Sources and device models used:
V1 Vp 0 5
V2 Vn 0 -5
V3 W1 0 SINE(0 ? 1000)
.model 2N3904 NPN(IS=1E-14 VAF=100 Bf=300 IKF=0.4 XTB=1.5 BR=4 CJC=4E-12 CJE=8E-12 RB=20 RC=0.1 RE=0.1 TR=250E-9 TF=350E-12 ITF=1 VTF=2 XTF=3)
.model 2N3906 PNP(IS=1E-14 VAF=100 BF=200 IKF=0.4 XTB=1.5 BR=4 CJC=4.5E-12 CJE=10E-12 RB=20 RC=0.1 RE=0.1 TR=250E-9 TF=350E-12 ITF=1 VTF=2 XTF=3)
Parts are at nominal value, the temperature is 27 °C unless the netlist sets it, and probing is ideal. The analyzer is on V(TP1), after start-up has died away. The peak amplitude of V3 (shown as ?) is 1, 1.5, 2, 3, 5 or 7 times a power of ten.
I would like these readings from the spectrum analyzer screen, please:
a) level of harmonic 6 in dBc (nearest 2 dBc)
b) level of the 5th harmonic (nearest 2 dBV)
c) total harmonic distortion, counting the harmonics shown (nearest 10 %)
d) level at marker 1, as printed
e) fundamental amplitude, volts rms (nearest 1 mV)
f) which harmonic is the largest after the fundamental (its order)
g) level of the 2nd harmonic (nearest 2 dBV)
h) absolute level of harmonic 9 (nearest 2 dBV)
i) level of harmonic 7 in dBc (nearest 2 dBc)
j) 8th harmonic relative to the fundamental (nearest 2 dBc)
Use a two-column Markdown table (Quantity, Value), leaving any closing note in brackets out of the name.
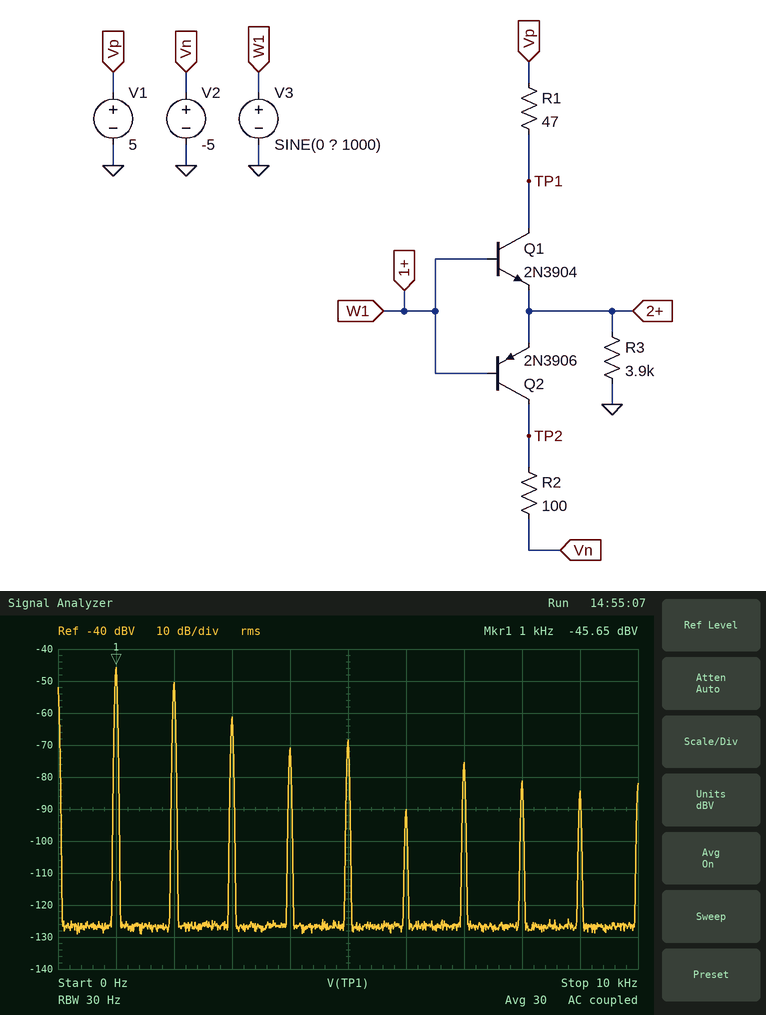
| Quantity | Value |
|---|---|
| level of harmonic 6 in dBc | -44 dBc |
| level of the 5th harmonic | -68 dBV |
| total harmonic distortion, counting the harmonics shown | 60 % |
| level at marker 1, as printed | -45.65 dBV |
| fundamental amplitude, volts rms | 5 mV |
| which harmonic is the largest after the fundamental | 2 |
| level of the 2nd harmonic | -50 dBV |
| absolute level of harmonic 9 | -84 dBV |
| level of harmonic 7 in dBc | -30 dBc |
| 8th harmonic relative to the fundamental | -36 dBc |
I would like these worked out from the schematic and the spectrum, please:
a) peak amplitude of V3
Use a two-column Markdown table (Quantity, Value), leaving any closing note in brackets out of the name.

| Quantity | Value |
|---|---|
| peak amplitude of V3 | 2 V |
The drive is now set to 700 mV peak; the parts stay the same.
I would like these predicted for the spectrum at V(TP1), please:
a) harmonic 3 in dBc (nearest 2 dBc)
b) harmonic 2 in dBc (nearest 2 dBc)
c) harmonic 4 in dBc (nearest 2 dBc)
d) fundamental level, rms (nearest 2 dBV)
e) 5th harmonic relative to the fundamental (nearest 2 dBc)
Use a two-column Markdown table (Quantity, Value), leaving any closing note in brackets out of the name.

| Quantity | Value |
|---|---|
| harmonic 3 in dBc | -4 dBc |
| harmonic 2 in dBc | -2 dBc |
| harmonic 4 in dBc | -8 dBc |
| fundamental level, rms | -70 dBV |
| 5th harmonic relative to the fundamental | -16 dBc |
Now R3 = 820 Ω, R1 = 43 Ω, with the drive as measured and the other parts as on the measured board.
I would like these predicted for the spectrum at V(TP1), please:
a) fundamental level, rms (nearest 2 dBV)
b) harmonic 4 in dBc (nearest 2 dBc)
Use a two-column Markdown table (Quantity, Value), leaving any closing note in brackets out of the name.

| Quantity | Value |
|---|---|
| fundamental level, rms | -34 dBV |
| harmonic 4 in dBc | -26 dBc |
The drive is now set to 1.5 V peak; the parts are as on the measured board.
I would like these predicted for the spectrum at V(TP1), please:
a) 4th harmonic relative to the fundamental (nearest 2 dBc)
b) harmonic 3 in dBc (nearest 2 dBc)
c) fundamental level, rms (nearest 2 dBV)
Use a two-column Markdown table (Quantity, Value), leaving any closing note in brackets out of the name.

| Quantity | Value |
|---|---|
| 4th harmonic relative to the fundamental | -36 dBc |
| harmonic 3 in dBc | -12 dBc |
| fundamental level, rms | -50 dBV |
